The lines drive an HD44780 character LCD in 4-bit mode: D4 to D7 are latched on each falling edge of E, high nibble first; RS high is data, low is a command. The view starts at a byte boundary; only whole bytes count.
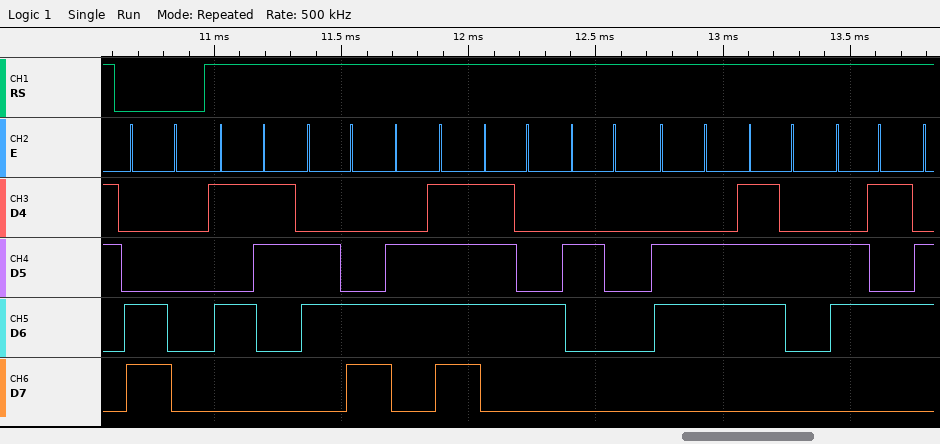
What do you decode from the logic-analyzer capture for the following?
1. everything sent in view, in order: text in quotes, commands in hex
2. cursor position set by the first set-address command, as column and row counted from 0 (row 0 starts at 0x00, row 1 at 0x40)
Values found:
0xC0 "Slot fre"
column 0, row 1
